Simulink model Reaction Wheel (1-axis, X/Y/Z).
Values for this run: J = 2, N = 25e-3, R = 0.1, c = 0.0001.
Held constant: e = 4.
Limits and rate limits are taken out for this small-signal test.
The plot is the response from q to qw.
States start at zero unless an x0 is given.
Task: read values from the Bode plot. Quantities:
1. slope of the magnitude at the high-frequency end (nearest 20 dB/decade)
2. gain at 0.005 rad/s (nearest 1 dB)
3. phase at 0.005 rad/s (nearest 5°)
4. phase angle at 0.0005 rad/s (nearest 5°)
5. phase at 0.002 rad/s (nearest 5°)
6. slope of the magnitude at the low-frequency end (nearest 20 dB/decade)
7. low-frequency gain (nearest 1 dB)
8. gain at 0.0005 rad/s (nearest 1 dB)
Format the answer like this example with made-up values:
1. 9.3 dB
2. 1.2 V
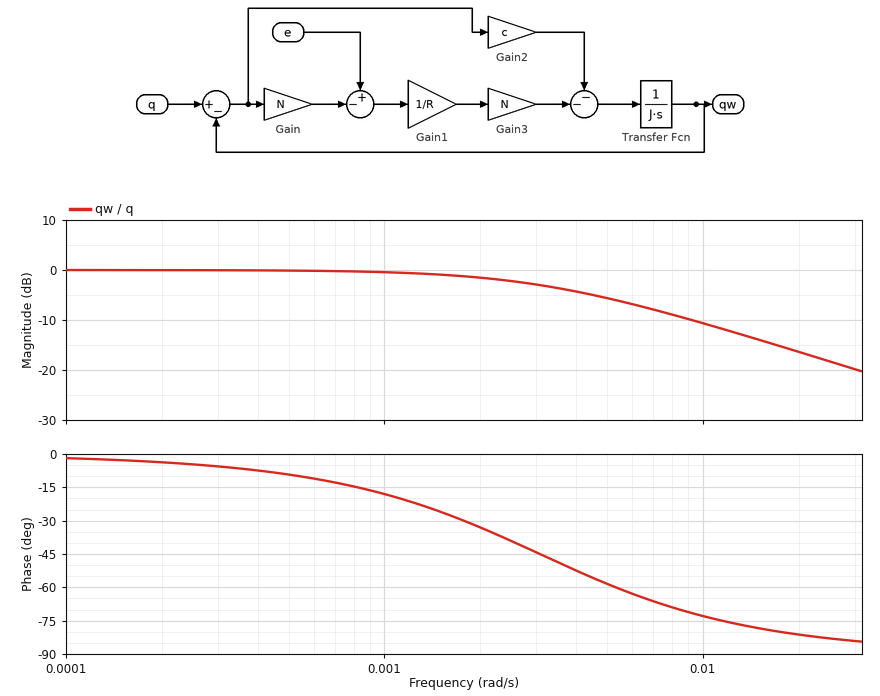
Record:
1. -20 dB/decade
2. -6 dB
3. -60°
4. -10°
5. -35°
6. 0 dB/decade
7. 0 dB
8. 0 dB
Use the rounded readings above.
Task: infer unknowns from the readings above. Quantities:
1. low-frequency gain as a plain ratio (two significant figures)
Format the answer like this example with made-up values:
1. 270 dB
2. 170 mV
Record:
1. 1.0
